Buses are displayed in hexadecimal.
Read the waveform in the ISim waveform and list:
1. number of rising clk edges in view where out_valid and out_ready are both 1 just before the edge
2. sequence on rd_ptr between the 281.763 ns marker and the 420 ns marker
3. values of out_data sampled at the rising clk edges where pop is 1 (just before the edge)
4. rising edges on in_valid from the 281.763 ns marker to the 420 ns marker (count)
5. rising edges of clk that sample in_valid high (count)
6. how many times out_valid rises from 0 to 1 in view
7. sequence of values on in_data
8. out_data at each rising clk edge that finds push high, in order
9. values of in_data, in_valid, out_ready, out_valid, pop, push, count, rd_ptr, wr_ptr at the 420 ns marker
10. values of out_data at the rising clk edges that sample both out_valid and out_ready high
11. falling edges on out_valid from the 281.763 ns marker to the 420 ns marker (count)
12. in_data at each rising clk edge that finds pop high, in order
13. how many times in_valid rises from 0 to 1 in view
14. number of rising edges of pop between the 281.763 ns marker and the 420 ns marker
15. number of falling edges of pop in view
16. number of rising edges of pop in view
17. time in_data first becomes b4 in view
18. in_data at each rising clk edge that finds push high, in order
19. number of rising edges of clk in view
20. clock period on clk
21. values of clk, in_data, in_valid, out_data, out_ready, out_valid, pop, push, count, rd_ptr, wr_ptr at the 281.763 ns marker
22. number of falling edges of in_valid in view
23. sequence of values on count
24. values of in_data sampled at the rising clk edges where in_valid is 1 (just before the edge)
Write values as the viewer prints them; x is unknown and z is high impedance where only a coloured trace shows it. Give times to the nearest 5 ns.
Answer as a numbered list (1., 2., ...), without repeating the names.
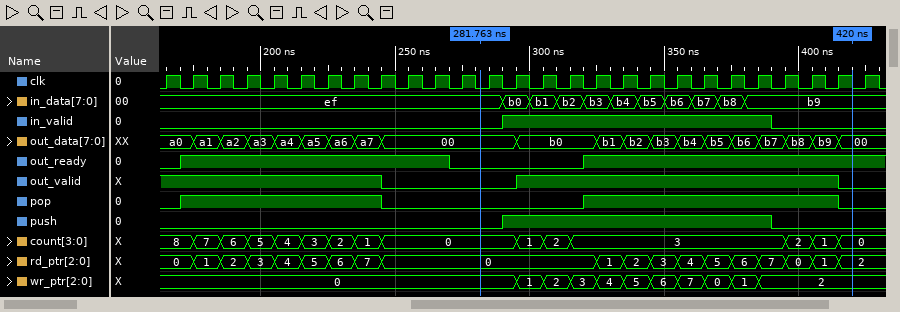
1. 18
2. 0, 1, 2, 3, 4, 5, 6, 7, 0, 1, 2
3. a0, a1, a2, a3, a4, a5, a6, a7, b0, b1, b2, b3, b4, b5, b6, b7, b8, b9
4. 1
5. 10
6. 1
7. ef, b0, b1, b2, b3, b4, b5, b6, b7, b8, b9
8. 00, b0, b0, b0, b1, b2, b3, b4, b5, b6
9. in_data=b9, in_valid=0, out_ready=1, out_valid=0, pop=0, push=0, count=0, rd_ptr=2, wr_ptr=2
10. a0, a1, a2, a3, a4, a5, a6, a7, b0, b1, b2, b3, b4, b5, b6, b7, b8, b9
11. 1
12. ef, ef, ef, ef, ef, ef, ef, ef, b3, b4, b5, b6, b7, b8, b9, b9, b9, b9
13. 1
14. 1
15. 2
16. 2
17. 330 ns
18. b0, b1, b2, b3, b4, b5, b6, b7, b8, b9
19. 27
20. 10 ns
21. clk=0, in_data=ef, in_valid=0, out_data=00, out_ready=0, out_valid=0, pop=0, push=0, count=0, rd_ptr=0, wr_ptr=0
22. 1
23. 8, 7, 6, 5, 4, 3, 2, 1, 0, 1, 2, 3, 2, 1, 0
24. b0, b1, b2, b3, b4, b5, b6, b7, b8, b9
